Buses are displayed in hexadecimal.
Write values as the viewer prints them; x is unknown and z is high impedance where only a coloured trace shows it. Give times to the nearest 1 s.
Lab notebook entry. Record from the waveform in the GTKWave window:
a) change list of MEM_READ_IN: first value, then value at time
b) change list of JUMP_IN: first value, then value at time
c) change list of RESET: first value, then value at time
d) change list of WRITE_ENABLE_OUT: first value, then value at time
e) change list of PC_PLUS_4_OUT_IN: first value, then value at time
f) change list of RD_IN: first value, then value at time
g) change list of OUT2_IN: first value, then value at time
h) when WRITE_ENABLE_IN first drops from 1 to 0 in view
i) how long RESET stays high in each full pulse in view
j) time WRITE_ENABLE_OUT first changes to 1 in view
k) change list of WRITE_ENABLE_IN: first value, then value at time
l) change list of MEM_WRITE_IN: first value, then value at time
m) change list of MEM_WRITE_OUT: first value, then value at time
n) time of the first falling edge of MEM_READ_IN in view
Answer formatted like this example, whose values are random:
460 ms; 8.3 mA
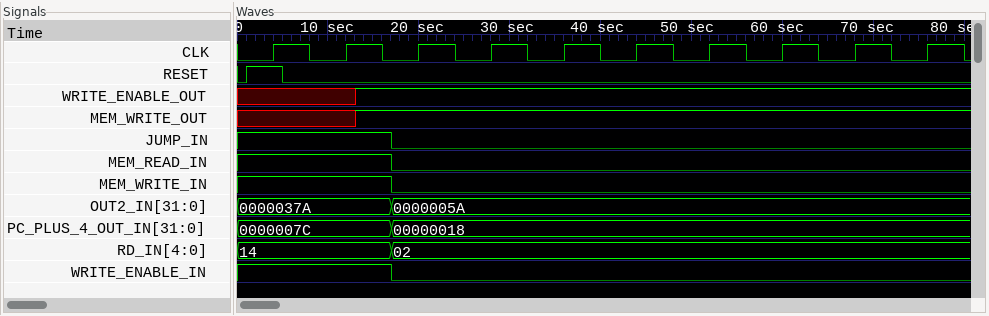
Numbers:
1, 0 at 17 s; 1, 0 at 17 s; 0, 1 at 1 s, 0 at 5 s; x, 1 at 13 s; 0000007C, 00000018 at 17 s; 14, 02 at 17 s; 0000037A, 0000005A at 17 s; 17 s; 4 s; 13 s; 1, 0 at 17 s; 1, 0 at 17 s; x, 1 at 13 s; 17 s
